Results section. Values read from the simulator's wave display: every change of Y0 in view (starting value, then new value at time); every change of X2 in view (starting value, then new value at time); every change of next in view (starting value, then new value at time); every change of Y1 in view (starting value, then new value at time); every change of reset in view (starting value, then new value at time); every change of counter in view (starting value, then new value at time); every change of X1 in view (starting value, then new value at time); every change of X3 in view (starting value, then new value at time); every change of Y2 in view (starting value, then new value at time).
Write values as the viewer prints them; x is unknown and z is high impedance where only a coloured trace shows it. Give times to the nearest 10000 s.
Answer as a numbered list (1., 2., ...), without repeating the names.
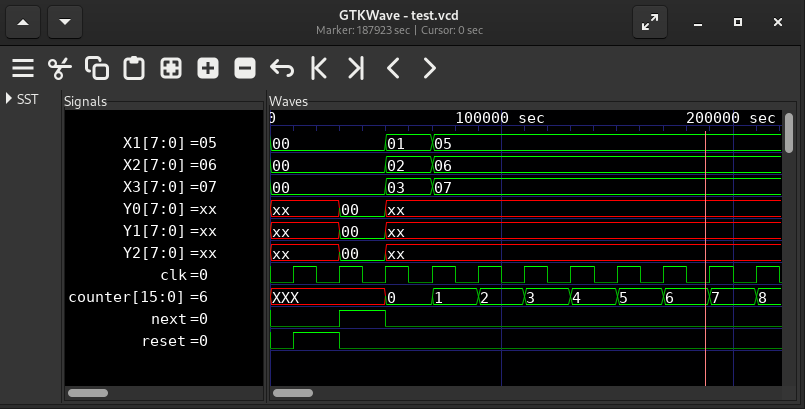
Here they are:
1. xx, 00 at 30000 s, xx at 50000 s
2. 00, 02 at 50000 s, 06 at 70000 s
3. 0, 1 at 30000 s, 0 at 50000 s
4. xx, 00 at 30000 s, xx at 50000 s
5. 0, 1 at 10000 s, 0 at 30000 s
6. XXX, 0 at 50000 s, 1 at 70000 s, 2 at 90000 s, 3 at 110000 s, 4 at 130000 s, 5 at 150000 s, 6 at 170000 s, 7 at 190000 s, 8 at 210000 s
7. 00, 01 at 50000 s, 05 at 70000 s
8. 00, 03 at 50000 s, 07 at 70000 s
9. xx, 00 at 30000 s, xx at 50000 s
